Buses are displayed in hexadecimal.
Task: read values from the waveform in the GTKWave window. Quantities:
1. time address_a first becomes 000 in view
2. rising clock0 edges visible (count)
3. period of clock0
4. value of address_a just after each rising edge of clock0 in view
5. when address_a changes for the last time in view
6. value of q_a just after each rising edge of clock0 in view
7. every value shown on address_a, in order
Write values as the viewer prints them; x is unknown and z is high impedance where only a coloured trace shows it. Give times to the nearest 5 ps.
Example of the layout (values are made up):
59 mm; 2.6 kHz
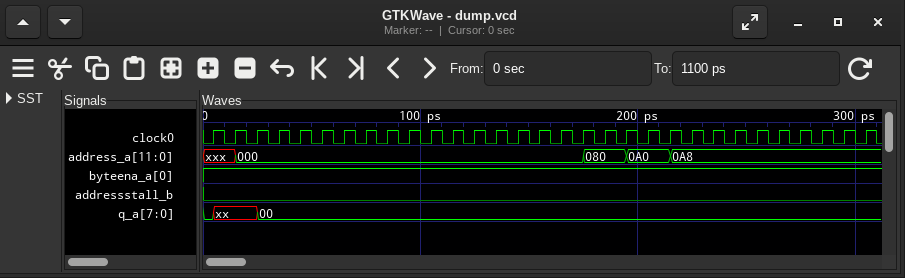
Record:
15 ps; 31; 10 ps; xxx, 000, 000, 000, 000, 000, 000, 000, 000, 000, 000, 000, 000, 000, 000, 000, 000, 080, 080, 0A0, 0A0, 0A8, 0A8, 0A8, 0A8, 0A8, 0A8, 0A8, 0A8, 0A8, 0A8; 215 ps; xx, xx, 00, 00, 00, 00, 00, 00, 00, 00, 00, 00, 00, 00, 00, 00, 00, 00, 00, 00, 00, 00, 00, 00, 00, 00, 00, 00, 00, 00, 00; xxx, 000, 080, 0A0, 0A8
